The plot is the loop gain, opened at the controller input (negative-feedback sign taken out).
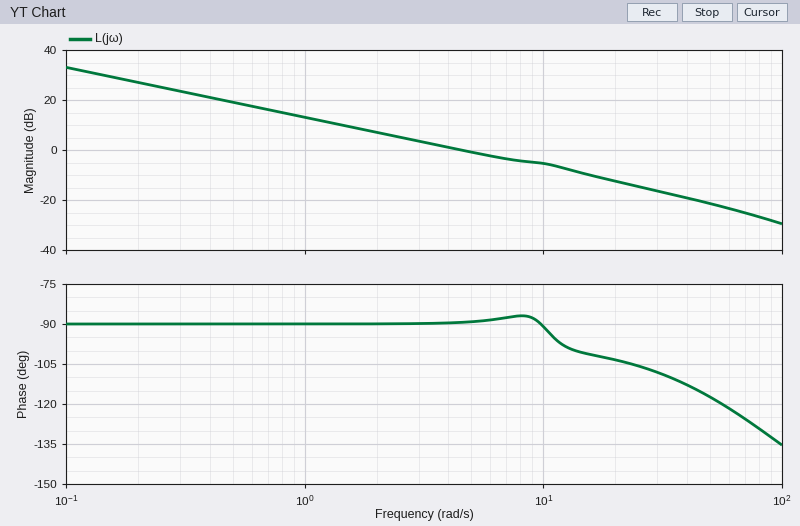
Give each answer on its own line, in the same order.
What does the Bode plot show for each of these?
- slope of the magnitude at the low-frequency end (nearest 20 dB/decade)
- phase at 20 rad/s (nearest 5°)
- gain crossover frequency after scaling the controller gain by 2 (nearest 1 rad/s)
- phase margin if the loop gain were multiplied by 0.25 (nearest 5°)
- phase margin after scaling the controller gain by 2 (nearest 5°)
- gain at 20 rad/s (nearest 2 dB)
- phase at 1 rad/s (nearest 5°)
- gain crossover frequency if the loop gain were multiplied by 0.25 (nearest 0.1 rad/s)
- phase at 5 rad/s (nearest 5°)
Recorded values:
-20 dB/decade
-105°
11 rad/s
90°
85°
-12 dB
-90°
1.1 rad/s
-90°
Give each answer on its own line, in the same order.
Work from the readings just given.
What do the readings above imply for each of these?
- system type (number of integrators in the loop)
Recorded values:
1
